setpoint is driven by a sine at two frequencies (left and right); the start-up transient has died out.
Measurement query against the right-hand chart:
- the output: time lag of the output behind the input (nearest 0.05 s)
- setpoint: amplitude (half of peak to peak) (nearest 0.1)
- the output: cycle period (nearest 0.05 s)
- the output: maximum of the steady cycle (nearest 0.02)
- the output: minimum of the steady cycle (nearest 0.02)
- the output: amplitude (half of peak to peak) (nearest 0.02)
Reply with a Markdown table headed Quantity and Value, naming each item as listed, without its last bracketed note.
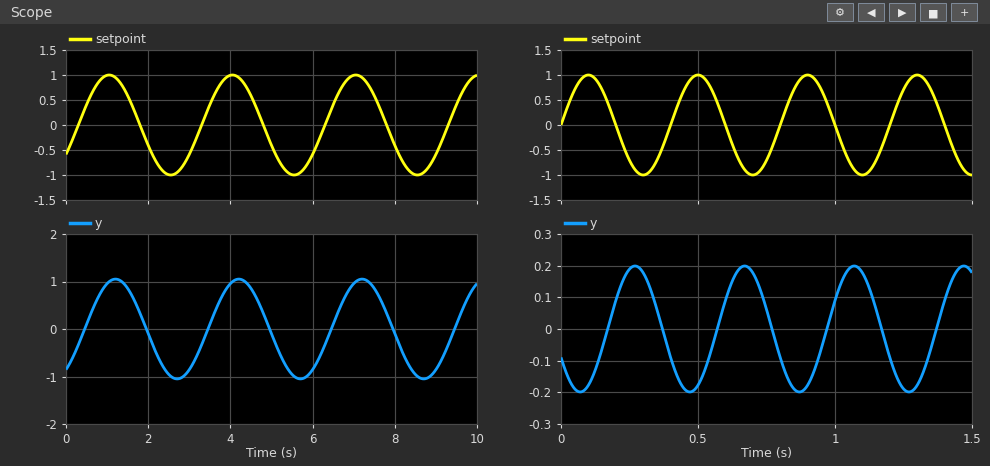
| Quantity | Value |
|---|---|
| the output: time lag of the output behind the input | 0.15 s |
| setpoint: amplitude (half of peak to peak) | 1.0 |
| the output: cycle period | 0.40 s |
| the output: maximum of the steady cycle | 0.20 |
| the output: minimum of the steady cycle | -0.20 |
| the output: amplitude (half of peak to peak) | 0.20 |
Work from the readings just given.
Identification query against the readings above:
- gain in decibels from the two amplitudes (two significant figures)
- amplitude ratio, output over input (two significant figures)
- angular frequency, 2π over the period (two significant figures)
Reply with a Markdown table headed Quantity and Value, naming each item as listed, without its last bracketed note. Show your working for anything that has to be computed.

| Quantity | Value |
|---|---|
| gain in decibels from the two amplitudes | 20 log10(0.2 / 1) = -14 dB |
| amplitude ratio, output over input | 0.2 / 1 = 0.20 |
| angular frequency, 2π over the period | 2π / 0.4 = 16 rad/s |
